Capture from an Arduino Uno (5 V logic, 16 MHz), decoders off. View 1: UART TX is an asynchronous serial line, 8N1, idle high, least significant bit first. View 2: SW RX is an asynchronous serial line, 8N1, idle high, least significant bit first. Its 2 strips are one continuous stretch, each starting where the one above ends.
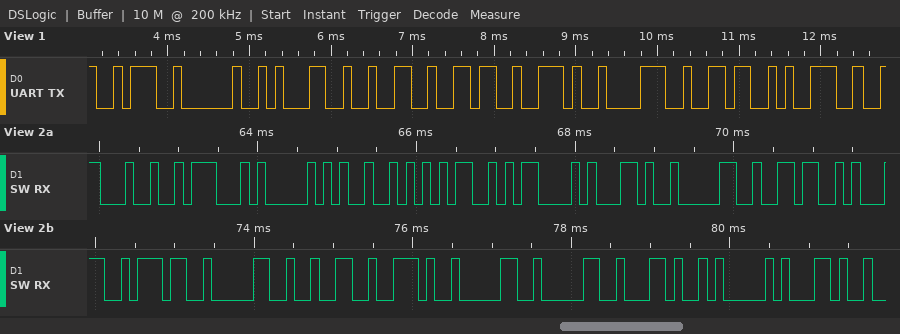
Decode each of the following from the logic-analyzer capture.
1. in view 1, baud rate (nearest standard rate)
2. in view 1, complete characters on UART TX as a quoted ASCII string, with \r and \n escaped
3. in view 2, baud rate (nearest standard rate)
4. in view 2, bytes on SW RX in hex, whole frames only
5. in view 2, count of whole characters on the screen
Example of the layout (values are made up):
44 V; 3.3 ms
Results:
9600 baud; ": 126.869"; 9600 baud; 24 47 50 52 4D 43 2C 30 36 31 37 30 32 2E 30 30 2C 41 2C; 19
